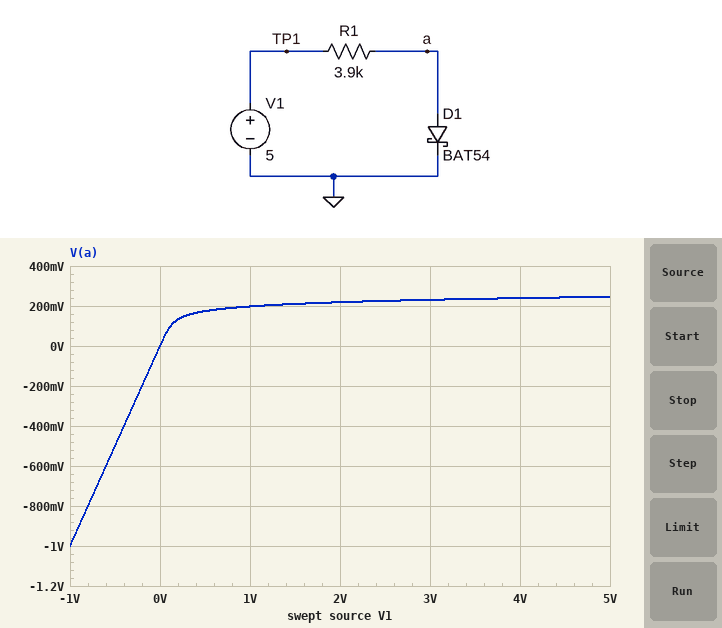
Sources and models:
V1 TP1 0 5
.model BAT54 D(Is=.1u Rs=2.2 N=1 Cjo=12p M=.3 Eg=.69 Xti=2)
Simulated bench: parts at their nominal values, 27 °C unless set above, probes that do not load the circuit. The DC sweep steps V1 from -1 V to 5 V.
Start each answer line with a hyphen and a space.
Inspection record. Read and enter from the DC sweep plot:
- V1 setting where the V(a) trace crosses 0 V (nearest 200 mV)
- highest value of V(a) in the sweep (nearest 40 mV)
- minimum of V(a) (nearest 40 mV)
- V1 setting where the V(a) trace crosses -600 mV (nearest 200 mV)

- 0 V
- 240 mV
- -1.00 V
- -600 mV
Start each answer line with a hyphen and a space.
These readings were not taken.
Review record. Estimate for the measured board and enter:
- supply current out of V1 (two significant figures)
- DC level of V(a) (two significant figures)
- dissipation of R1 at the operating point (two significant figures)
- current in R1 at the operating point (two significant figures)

- 1.2 mA
- 250 mV
- 5.8 mW
- 1.2 mA
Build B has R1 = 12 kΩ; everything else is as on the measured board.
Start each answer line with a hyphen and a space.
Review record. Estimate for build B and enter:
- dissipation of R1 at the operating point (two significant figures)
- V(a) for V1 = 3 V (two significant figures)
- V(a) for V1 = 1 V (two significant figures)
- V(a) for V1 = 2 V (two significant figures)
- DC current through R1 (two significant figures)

- 1.9 mW
- 200 mV
- 170 mV
- 190 mV
- 400 µA
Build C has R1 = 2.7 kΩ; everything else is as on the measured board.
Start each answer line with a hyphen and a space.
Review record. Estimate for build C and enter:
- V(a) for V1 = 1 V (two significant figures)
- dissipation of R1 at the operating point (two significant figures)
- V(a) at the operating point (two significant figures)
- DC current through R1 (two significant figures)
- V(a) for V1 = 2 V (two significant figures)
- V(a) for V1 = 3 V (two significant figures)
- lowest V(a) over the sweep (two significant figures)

- 210 mV
- 8.3 mW
- 260 mV
- 1.8 mA
- 230 mV
- 240 mV
- -1.0 V
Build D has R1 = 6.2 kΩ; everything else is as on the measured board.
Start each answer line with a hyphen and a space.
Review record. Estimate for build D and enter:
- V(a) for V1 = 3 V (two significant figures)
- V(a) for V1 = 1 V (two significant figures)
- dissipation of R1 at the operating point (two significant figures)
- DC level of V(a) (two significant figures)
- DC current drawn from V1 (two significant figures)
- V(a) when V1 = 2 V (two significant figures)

- 220 mV
- 190 mV
- 3.7 mW
- 230 mV
- 770 µA
- 210 mV
